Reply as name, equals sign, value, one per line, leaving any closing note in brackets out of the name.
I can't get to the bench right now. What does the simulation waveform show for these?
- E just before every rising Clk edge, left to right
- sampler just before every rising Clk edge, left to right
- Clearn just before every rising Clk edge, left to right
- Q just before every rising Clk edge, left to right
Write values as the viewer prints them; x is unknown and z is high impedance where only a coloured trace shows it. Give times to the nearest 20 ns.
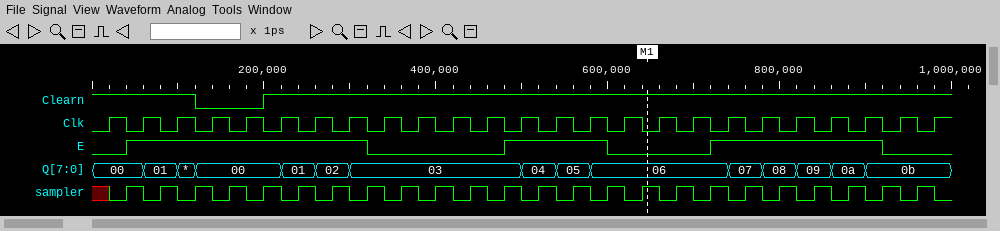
E just before every rising Clk edge, left to right = 0 1 1 1 1 1 1 1 0 0 0 0 1 1 1 0 0 0 1 1 1 1 1 0 0
sampler just before every rising Clk edge, left to right = x 1 1 1 1 1 1 1 1 1 1 1 1 1 1 1 1 1 1 1 1 1 1 1 1
Clearn just before every rising Clk edge, left to right = 1 1 1 0 0 1 1 1 1 1 1 1 1 1 1 1 1 1 1 1 1 1 1 1 1
Q just before every rising Clk edge, left to right = 00, 00, 01, 00, 00, 00, 01, 02, 03, 03, 03, 03, 03, 04, 05, 06, 06, 06, 06, 07, 08, 09, 0a, 0b, 0b
